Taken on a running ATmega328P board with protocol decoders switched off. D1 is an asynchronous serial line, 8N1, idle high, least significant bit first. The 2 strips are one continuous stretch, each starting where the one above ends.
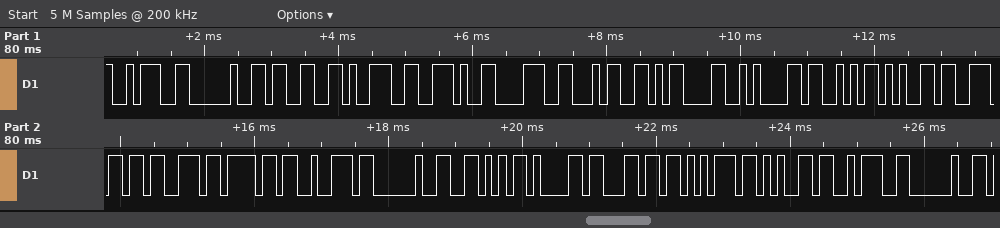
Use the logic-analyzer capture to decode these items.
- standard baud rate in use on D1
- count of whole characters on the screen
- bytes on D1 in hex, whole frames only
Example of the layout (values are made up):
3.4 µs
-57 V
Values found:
9600 baud
23
3A 20 33 39 2E 38 34 0D 0A 53 65 6E 73 6F 72 20 56 61 6C 75 65 3A 20
